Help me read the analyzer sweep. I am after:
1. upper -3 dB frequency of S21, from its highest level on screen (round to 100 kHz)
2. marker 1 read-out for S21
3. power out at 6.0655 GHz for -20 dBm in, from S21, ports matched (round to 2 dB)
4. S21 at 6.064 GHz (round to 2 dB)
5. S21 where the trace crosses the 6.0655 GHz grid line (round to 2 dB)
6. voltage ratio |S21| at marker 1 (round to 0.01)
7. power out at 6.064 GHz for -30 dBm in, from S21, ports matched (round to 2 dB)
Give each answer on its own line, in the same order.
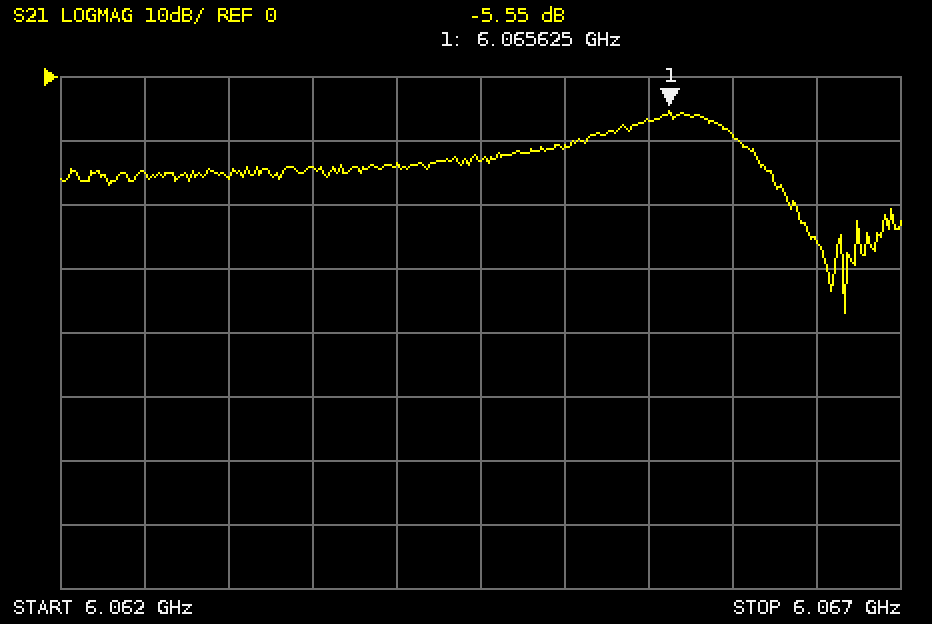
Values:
6.0660 GHz
-5.55 dB
-26 dBm
-14 dB
-6 dB
0.53
-44 dBm
